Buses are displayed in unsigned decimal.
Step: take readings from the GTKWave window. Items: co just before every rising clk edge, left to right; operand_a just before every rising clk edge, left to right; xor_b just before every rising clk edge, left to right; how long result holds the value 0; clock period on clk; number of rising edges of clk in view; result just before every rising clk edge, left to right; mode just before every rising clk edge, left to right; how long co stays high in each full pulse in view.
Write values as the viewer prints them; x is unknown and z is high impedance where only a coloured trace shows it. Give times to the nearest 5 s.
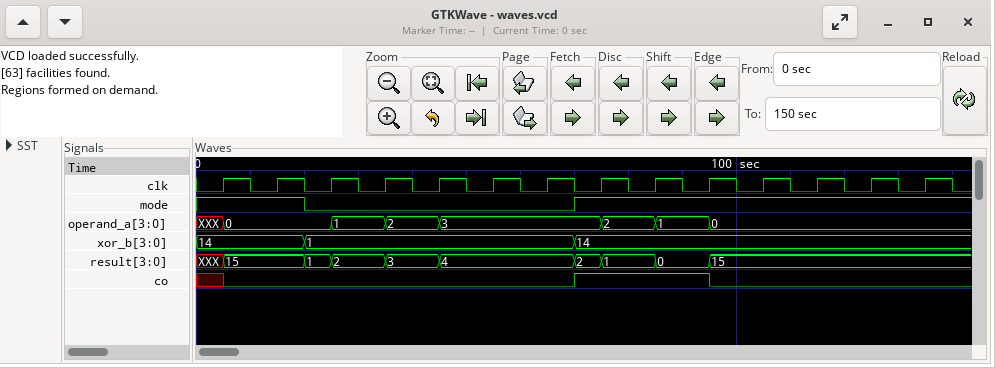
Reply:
x 0 0 0 0 0 0 1 1 1 0 0 0 0
XXX, 0, 0, 1, 2, 3, 3, 3, 2, 1, 0, 0, 0, 0
14, 14, 1, 1, 1, 1, 1, 14, 14, 14, 14, 14, 14, 14
10 s
10 s
14
XXX, 15, 1, 2, 3, 4, 4, 2, 1, 0, 15, 15, 15, 15
1 1 0 0 0 0 0 1 1 1 1 1 1 1
25 s
